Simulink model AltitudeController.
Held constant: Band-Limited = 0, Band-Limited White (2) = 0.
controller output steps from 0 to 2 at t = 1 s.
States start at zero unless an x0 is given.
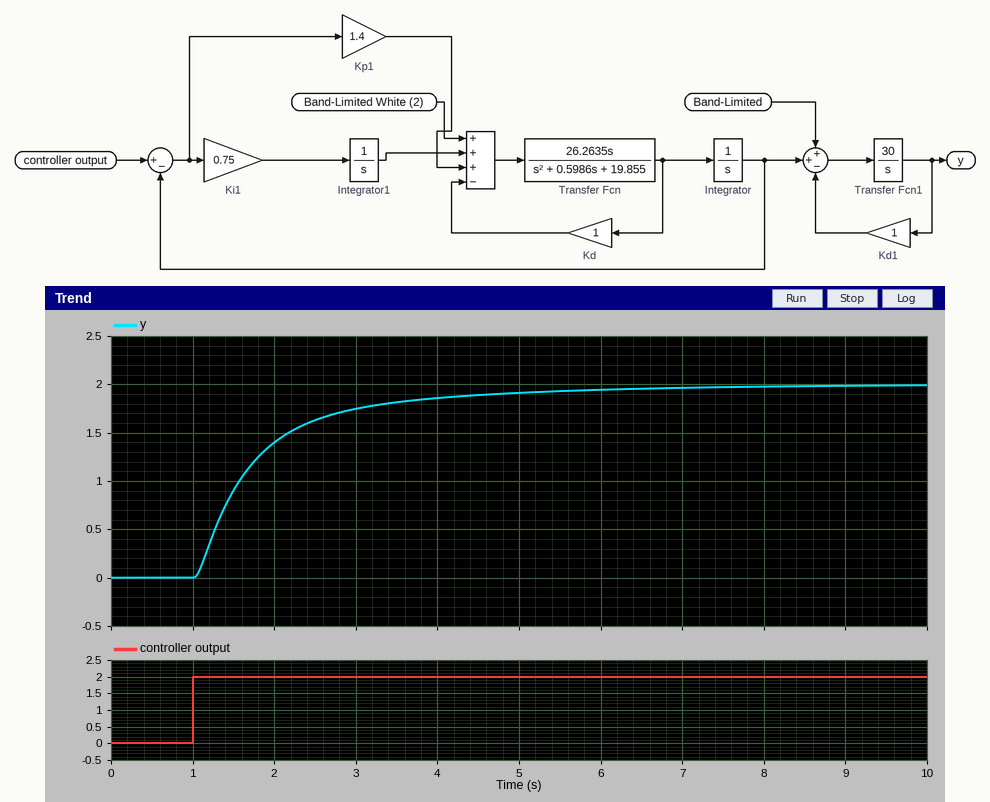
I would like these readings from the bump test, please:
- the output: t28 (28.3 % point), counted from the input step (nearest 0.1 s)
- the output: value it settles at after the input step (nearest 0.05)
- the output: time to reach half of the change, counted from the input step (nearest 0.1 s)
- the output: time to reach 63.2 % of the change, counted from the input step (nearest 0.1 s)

0.3 s
2.00
0.6 s
0.8 s
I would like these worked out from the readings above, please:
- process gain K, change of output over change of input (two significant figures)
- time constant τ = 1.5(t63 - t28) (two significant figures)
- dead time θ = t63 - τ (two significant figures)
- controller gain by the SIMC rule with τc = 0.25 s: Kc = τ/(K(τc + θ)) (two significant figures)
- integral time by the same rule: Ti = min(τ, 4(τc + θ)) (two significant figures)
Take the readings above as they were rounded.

1.0
0.75 s
0.050 s
2.5
0.75 s
